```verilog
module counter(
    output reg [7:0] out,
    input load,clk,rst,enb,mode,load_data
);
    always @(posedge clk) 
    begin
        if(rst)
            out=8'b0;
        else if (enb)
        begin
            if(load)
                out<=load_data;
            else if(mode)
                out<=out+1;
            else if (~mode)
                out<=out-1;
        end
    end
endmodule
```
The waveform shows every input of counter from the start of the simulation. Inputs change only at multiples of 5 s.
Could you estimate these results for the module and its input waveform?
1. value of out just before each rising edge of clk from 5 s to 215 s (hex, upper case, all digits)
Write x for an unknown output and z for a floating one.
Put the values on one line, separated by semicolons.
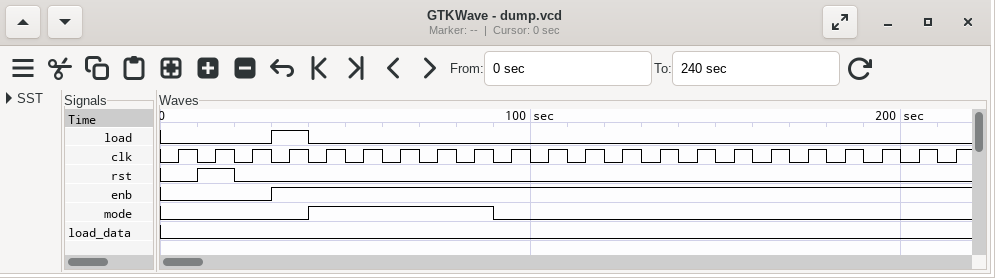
x, x, 00, 00, 00, 01, 02, 03, 04, 05, 04, 03, 02, 01, 00, FF, FE, FD, FC, FB, FA, F9
